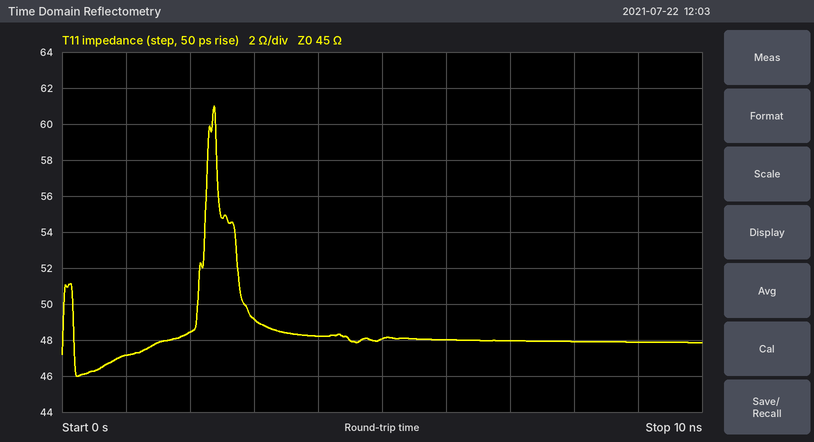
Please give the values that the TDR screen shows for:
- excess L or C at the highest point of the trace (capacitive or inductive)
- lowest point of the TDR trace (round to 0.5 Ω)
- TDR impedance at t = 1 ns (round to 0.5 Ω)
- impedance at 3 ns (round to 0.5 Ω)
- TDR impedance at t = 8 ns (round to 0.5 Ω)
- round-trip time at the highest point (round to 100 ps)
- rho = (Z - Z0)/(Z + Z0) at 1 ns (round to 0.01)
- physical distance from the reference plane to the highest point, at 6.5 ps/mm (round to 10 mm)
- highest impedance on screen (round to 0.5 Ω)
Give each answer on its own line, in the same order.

inductive
46.0 Ω
47.0 Ω
49.0 Ω
48.0 Ω
2.4 ns
+0.02
180 mm
61.0 Ω
